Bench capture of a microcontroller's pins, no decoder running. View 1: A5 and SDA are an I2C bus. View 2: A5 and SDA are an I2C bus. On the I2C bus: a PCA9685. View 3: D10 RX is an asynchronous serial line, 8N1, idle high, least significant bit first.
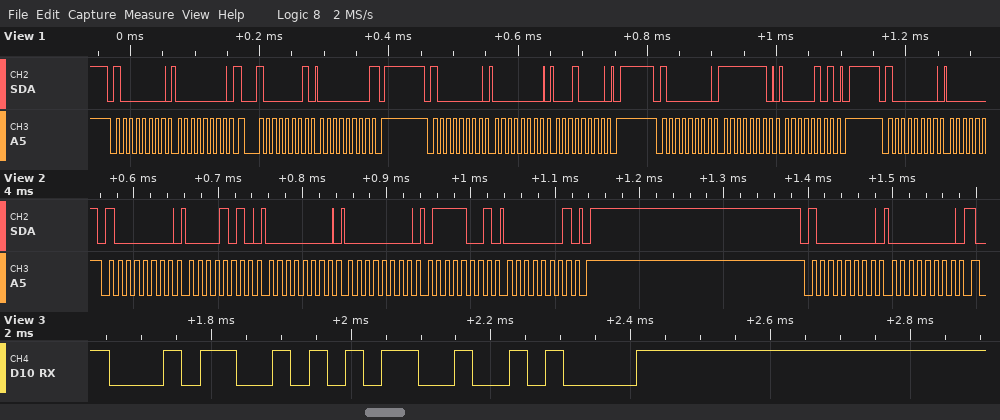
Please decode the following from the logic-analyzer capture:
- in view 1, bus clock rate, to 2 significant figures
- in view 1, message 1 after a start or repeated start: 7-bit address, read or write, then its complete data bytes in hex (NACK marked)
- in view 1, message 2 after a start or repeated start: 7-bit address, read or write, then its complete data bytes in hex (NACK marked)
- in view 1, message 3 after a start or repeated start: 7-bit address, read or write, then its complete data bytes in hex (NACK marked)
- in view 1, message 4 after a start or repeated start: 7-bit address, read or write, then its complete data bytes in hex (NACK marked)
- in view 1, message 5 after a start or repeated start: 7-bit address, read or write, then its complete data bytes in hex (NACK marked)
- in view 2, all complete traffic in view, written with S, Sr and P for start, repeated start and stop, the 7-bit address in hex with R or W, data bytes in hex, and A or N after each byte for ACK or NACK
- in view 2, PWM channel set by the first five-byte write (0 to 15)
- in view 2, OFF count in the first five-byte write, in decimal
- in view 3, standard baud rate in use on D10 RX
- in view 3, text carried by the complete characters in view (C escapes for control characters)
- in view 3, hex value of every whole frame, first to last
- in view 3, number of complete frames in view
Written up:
100 kHz
0x40 write: 00
0x40 read: 00 NACK
0x40 write: 00 10
0x40 write: FE 05
0x40 write
S 40W A 0A A 00 A 00 A 79 A 01 A P S 40W A 00 A
1
377
38400 baud
"45\n"
34 35 0A
3
